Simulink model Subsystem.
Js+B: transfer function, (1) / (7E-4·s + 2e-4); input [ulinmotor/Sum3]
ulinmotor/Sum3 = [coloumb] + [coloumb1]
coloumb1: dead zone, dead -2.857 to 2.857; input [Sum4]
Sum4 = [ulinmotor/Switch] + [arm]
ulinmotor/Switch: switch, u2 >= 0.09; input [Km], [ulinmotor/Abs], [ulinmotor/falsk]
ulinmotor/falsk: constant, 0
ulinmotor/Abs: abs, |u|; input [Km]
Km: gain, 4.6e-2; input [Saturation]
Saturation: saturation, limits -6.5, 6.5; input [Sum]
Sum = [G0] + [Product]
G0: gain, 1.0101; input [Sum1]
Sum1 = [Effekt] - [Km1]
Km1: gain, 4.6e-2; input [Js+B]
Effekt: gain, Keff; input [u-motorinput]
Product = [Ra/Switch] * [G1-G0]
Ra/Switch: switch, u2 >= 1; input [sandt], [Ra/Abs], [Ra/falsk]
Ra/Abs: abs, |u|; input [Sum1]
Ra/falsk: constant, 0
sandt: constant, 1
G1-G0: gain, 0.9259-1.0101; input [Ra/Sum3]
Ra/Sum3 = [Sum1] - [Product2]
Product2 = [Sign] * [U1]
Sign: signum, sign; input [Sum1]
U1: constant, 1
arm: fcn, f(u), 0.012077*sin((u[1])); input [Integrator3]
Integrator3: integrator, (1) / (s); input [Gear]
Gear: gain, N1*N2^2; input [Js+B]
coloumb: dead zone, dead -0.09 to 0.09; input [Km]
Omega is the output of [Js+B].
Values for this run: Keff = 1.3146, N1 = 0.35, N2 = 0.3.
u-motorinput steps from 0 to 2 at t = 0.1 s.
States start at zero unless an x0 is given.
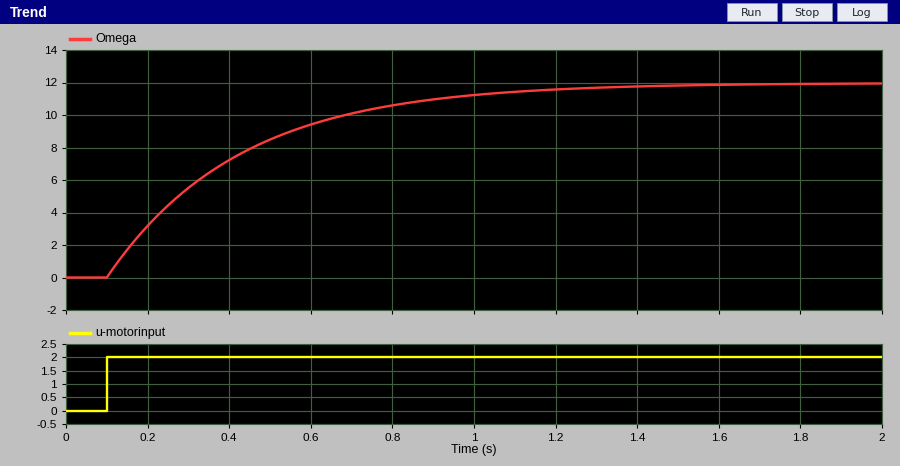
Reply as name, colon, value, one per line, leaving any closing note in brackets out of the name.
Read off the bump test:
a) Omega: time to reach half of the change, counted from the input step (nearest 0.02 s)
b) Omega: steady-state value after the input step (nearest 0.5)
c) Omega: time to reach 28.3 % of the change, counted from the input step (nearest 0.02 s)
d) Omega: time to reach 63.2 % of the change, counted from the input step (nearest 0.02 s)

Omega: time to reach half of the change, counted from the input step: 0.22 s
Omega: steady-state value after the input step: 12.0
Omega: time to reach 28.3 % of the change, counted from the input step: 0.10 s
Omega: time to reach 63.2 % of the change, counted from the input step: 0.32 s
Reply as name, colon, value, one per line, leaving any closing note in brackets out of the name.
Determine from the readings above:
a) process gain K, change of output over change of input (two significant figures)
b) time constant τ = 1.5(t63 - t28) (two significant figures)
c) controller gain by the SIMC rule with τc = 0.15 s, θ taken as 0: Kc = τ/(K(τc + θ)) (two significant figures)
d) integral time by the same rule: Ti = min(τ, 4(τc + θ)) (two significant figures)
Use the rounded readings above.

process gain K, change of output over change of input: 6.0
time constant τ = 1.5(t63 - t28): 0.33 s
controller gain by the SIMC rule with τc = 0.15 s, θ taken as 0: Kc = τ/(K(τc + θ)): 0.37
integral time by the same rule: Ti = min(τ, 4(τc + θ)): 0.33 s
